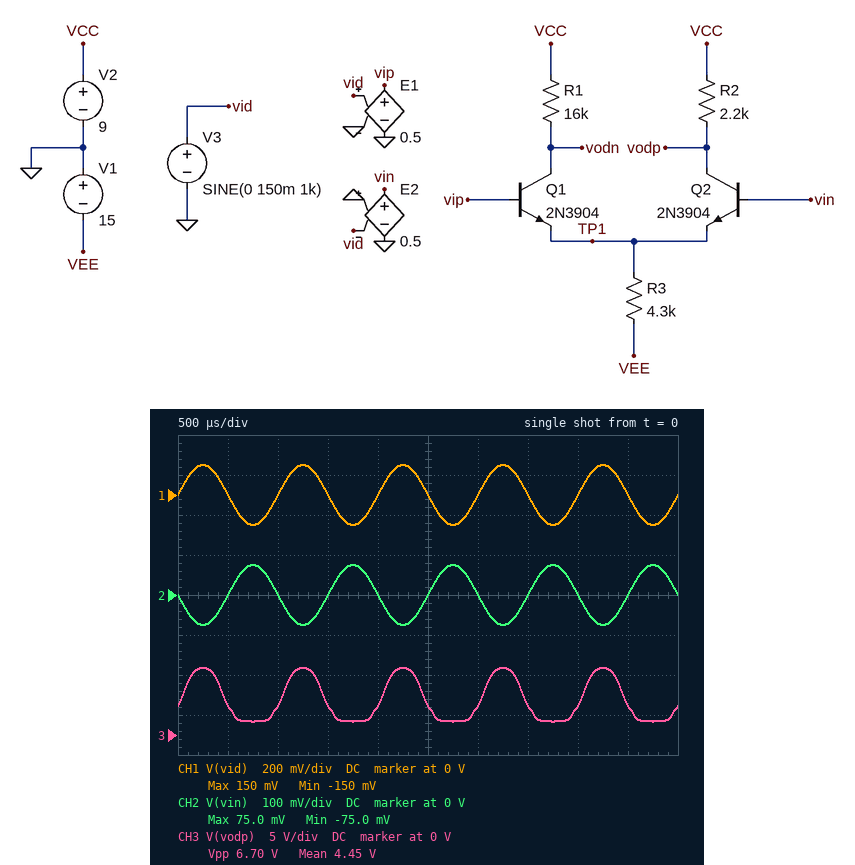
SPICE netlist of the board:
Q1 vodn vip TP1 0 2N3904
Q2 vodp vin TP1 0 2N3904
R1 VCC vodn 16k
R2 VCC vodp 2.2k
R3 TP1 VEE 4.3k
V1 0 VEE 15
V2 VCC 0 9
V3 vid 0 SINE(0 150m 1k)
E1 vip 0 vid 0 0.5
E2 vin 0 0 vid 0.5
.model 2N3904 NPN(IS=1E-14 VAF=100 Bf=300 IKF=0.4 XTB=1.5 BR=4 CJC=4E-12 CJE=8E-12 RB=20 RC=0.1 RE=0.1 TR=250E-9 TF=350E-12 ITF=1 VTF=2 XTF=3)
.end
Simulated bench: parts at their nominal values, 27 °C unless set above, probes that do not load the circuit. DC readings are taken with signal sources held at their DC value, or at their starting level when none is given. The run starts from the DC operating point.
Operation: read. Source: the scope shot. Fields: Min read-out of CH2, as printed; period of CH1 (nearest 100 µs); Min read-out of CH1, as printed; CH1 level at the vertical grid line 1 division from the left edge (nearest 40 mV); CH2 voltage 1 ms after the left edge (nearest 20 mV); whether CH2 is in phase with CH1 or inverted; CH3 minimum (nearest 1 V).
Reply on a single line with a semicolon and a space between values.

-75.0 mV; 1.0 ms; -150 mV; 0 V; 0 V; inverted; 2 V
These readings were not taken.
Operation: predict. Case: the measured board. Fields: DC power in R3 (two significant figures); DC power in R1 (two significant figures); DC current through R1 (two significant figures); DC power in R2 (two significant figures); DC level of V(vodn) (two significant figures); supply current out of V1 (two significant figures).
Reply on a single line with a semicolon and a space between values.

48 mW; 5.8 mW; 600 µA; 13 mW; -660 mV; 3.3 mA
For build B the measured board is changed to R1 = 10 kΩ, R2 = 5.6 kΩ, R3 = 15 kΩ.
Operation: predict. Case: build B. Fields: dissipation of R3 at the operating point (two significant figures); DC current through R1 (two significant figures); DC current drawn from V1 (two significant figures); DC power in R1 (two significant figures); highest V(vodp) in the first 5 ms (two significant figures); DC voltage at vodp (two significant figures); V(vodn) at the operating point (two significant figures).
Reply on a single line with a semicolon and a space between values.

14 mW; 470 µA; 960 µA; 2.2 mW; 9.0 V; 6.3 V; 4.3 V
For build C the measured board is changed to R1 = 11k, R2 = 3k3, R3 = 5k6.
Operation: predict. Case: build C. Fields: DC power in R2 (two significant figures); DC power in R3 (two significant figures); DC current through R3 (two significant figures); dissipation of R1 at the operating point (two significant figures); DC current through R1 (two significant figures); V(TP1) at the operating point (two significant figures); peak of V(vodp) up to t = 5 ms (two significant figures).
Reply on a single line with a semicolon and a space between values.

8.1 mW; 37 mW; 2.6 mA; 8.4 mW; 880 µA; -670 mV; 8.7 V
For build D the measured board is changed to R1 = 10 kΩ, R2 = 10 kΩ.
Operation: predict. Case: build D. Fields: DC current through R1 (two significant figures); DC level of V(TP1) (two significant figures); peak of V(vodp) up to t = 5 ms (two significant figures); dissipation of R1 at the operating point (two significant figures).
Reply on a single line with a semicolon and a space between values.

970 µA; -710 mV; 7.0 V; 9.4 mW
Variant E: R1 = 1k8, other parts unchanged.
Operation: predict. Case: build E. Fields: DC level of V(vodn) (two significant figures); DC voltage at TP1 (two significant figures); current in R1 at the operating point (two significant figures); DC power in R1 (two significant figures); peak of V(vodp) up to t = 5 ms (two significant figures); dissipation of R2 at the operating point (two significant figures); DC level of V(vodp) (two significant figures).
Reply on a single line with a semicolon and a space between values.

6.0 V; -670 mV; 1.7 mA; 5.0 mW; 9.0 V; 6.0 mW; 5.4 V
